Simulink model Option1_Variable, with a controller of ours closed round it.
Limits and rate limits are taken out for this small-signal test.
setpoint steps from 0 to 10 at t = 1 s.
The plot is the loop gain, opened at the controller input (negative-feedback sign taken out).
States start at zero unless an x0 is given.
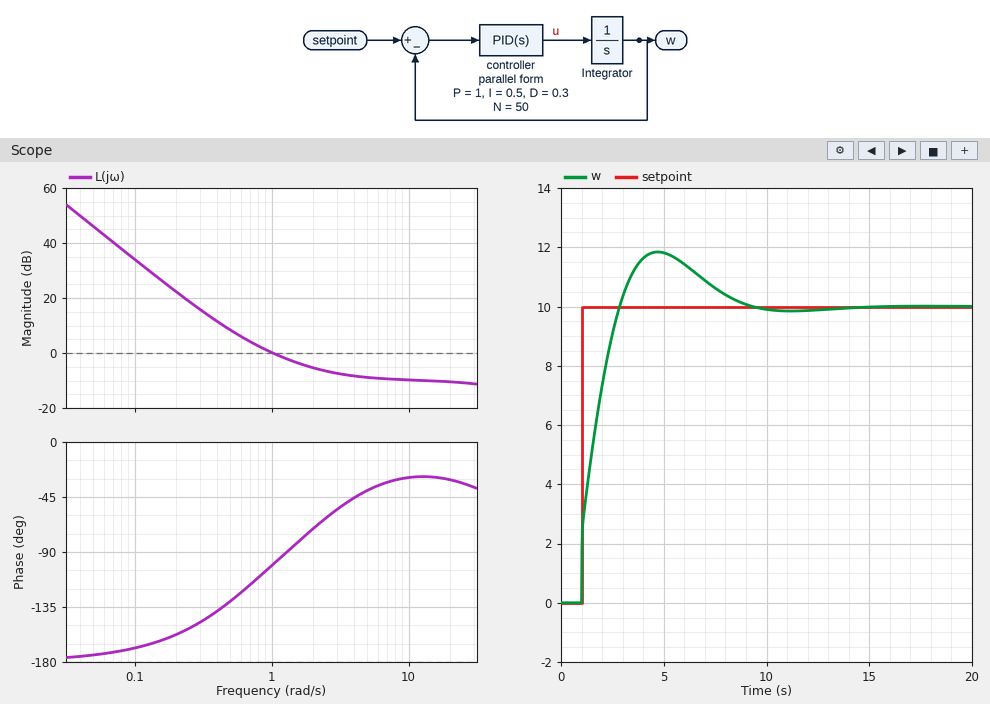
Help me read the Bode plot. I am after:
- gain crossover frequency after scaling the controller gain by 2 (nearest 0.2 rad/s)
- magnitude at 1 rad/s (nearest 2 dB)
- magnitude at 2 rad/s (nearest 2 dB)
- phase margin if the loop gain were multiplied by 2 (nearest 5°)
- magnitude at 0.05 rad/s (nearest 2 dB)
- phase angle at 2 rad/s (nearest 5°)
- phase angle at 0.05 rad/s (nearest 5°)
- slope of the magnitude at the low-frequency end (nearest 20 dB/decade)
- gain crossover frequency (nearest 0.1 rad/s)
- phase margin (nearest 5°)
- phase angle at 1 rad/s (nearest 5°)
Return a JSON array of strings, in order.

["2.2 rad/s", "0 dB", "-6 dB", "115°", "46 dB", "-70°", "-175°", "-40 dB/decade", "1.0 rad/s", "80°", "-100°"]
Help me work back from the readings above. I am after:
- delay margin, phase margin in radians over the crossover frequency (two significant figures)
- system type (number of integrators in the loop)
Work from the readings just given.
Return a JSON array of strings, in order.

["1.4 s", "2"]
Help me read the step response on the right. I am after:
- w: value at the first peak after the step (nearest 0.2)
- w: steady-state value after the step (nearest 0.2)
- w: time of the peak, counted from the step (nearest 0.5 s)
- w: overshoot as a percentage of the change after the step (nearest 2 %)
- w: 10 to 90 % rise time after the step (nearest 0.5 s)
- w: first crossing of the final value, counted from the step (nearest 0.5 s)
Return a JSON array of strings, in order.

["11.8", "10.0", "3.5 s", "18 %", "1.5 s", "2.0 s"]
